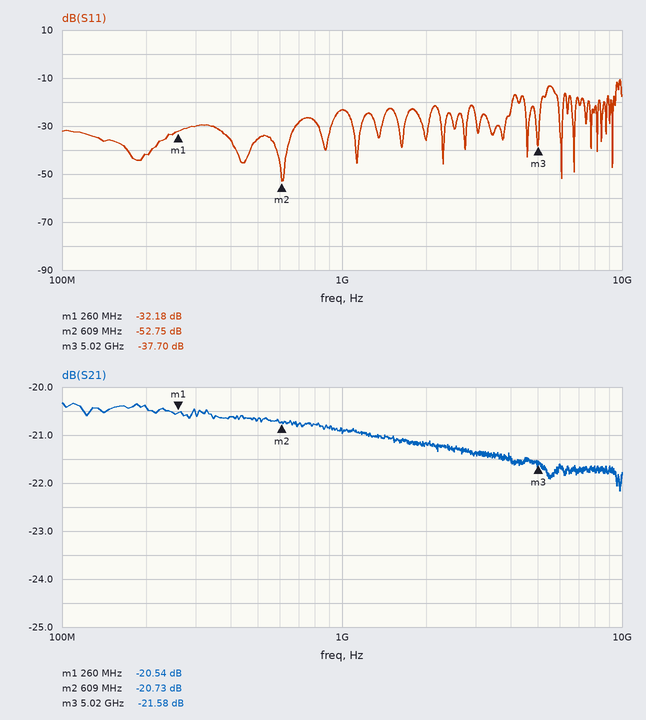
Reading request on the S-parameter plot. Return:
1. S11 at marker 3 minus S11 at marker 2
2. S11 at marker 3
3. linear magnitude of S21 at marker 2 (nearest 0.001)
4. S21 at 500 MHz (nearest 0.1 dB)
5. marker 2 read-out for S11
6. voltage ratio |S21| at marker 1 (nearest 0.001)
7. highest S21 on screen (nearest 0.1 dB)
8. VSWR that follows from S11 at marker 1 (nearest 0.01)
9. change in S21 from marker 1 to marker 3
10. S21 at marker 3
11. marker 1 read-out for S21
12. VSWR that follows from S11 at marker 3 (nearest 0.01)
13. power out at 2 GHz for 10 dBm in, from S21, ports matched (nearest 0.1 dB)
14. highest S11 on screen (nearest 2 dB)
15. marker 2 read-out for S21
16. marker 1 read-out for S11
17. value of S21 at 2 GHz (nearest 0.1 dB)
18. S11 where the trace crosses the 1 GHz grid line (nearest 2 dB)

15.05 dB
-37.70 dB
0.092
-20.7 dB
-52.75 dB
0.094
-20.3 dB
1.05
-1.04 dB
-21.58 dB
-20.54 dB
1.03
-11.2 dBm
-10 dB
-20.73 dB
-32.18 dB
-21.2 dB
-24 dB
